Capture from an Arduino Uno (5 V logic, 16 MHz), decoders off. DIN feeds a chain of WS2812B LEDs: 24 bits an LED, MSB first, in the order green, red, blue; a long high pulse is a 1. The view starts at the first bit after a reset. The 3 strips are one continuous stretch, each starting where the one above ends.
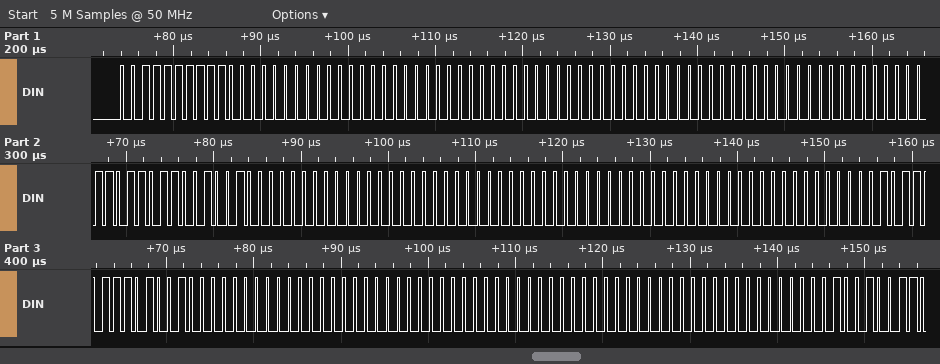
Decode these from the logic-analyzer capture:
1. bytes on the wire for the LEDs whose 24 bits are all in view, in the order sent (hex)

3F C0 00 00 00 00 00 00 00 36 C9 00 00 00 00 00 00 00 2D D2 00 00 00 00 00 00 00
